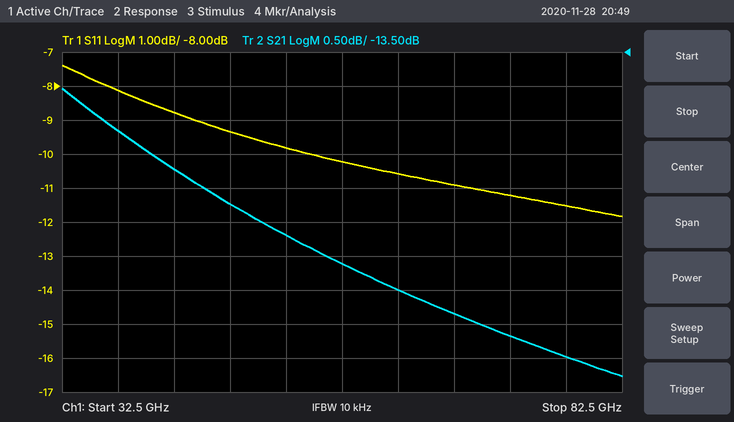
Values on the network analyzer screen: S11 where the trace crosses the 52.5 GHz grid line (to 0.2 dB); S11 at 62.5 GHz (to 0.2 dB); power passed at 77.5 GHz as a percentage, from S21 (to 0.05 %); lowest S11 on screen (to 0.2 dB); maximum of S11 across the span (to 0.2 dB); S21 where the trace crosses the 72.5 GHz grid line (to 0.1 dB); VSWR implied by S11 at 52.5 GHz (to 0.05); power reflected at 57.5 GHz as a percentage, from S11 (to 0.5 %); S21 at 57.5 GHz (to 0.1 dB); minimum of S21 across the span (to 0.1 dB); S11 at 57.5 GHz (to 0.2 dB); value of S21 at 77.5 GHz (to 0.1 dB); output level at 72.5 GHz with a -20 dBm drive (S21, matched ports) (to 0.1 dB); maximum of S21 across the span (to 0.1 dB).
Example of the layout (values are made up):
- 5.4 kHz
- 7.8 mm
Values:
- -9.8 dB
- -10.6 dB
- 1.60 %
- -11.8 dB
- -7.4 dB
- -17.7 dB
- 1.95
- 9.5 %
- -16.6 dB
- -18.3 dB
- -10.2 dB
- -18.0 dB
- -37.7 dBm
- -14.0 dB
